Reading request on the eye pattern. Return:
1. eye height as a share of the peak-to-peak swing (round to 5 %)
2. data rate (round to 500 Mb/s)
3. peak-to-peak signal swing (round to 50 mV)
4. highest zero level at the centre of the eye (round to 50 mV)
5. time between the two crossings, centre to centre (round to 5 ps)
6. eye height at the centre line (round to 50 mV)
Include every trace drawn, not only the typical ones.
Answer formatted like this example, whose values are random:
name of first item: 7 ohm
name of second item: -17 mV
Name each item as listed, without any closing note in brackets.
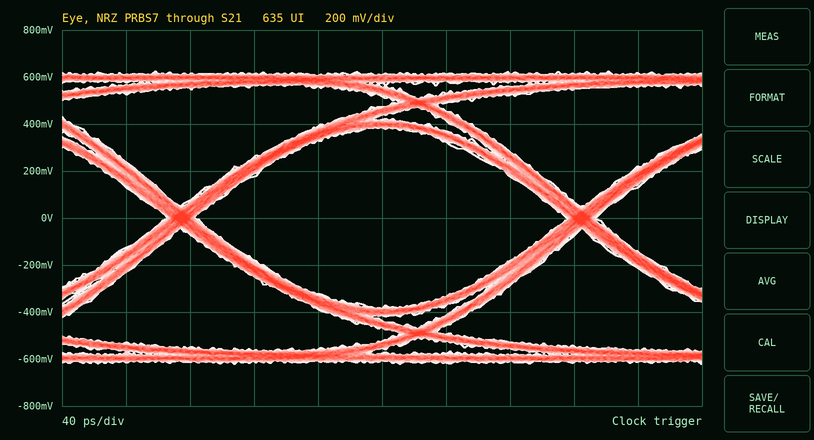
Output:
eye height as a share of the peak-to-peak swing: 60 %
data rate: 4.0 Gb/s
peak-to-peak signal swing: 1.25 V
highest zero level at the centre of the eye: -400 mV
time between the two crossings, centre to centre: 250 ps
eye height at the centre line: 750 mV
